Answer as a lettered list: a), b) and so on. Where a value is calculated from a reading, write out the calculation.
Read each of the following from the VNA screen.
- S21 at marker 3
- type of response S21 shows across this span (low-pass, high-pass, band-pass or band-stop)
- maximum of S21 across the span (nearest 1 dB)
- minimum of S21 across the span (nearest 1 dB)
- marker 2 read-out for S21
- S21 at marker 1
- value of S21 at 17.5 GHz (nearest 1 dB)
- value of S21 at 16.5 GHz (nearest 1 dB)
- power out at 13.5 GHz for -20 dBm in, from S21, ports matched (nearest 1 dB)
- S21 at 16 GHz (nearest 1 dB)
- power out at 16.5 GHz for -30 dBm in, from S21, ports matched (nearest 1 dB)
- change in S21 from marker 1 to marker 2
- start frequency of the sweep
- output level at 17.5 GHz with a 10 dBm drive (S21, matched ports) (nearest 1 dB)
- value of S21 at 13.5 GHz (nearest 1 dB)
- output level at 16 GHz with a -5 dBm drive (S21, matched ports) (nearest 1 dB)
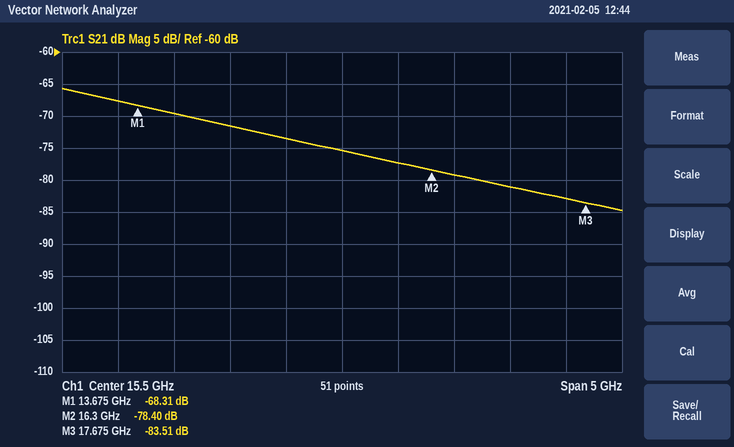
a) -83.51 dB
b) low-pass
c) -66 dB
d) -85 dB
e) -78.40 dB
f) -68.31 dB
g) -83 dB
h) -79 dB
i) -20 dBm + (-68 dB) = -88 dBm
j) -77 dB
k) -30 dBm + (-79 dB) = -109 dBm
l) -78.4 − (-68.31) = -10.09 dB
m) 13 GHz
n) 10 dBm + (-83 dB) = -73 dBm
o) -68 dB
p) -5 dBm + (-77 dB) = -82 dBm
